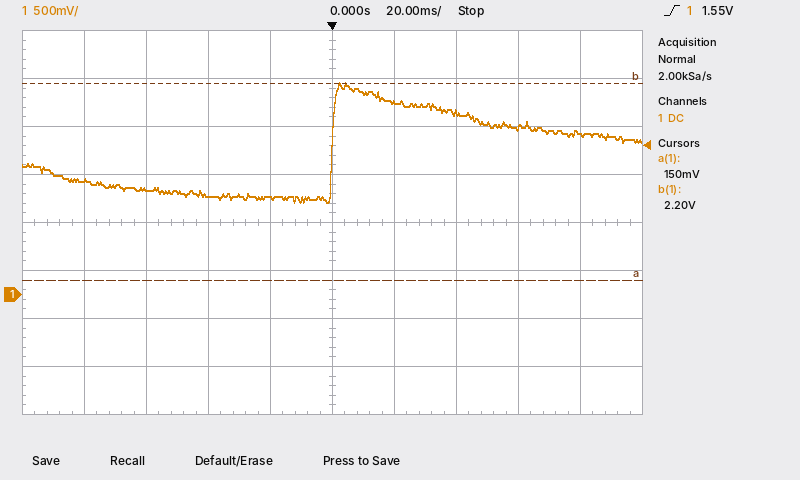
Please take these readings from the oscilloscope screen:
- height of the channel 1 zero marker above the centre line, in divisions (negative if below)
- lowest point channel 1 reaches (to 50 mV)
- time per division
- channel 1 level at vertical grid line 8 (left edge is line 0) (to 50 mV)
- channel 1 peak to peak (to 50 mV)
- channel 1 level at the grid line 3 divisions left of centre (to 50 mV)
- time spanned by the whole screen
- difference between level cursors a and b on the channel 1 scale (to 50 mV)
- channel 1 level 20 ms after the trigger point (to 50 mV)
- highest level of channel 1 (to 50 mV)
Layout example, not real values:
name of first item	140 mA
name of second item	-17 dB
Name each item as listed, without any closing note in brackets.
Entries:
height of the channel 1 zero marker above the centre line, in divisions	-1.5 div
lowest point channel 1 reaches	950 mV
time per division	20 ms
channel 1 level at vertical grid line 8 (left edge is line 0)	1.75 V
channel 1 peak to peak	1.25 V
channel 1 level at the grid line 3 divisions left of centre	1.10 V
time spanned by the whole screen	200 ms
difference between level cursors a and b on the channel 1 scale	2.05 V
channel 1 level 20 ms after the trigger point	2.00 V
highest level of channel 1	2.20 V
